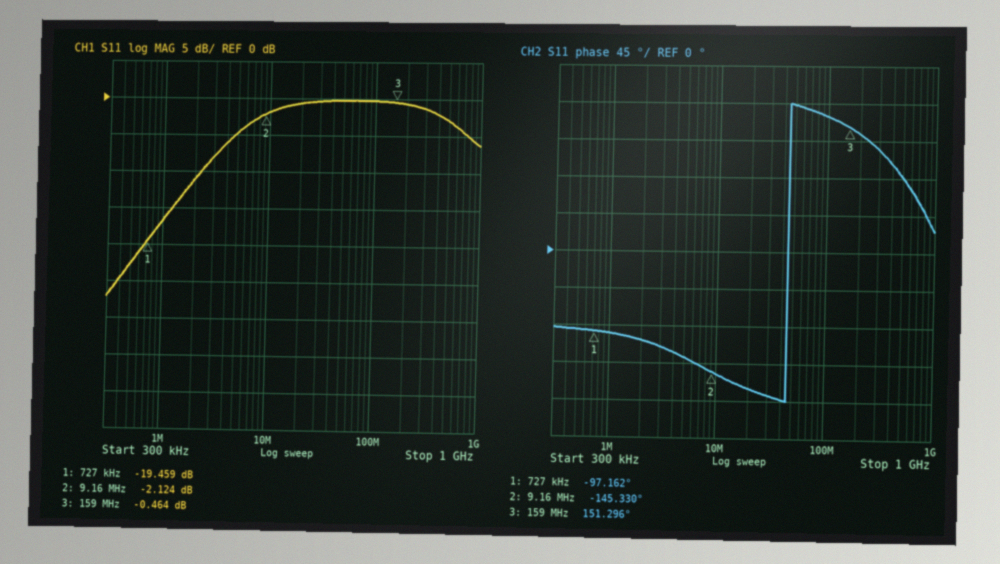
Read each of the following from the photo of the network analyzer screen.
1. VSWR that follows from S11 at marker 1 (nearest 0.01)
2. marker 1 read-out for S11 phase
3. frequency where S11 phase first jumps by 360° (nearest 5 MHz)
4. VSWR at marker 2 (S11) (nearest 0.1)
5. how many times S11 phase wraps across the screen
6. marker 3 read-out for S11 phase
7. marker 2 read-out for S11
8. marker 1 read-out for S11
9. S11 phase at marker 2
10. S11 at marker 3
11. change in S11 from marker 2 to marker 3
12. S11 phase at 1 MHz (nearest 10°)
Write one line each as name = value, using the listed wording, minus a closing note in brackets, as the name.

VSWR that follows from S11 at marker 1 = 1.24
marker 1 read-out for S11 phase = -97.162°
frequency where S11 phase first jumps by 360° = 45 MHz
VSWR at marker 2 (S11) = 8.2
how many times S11 phase wraps across the screen = 1
marker 3 read-out for S11 phase = 151.296°
marker 2 read-out for S11 = -2.124 dB
marker 1 read-out for S11 = -19.459 dB
S11 phase at marker 2 = -145.330°
S11 at marker 3 = -0.464 dB
change in S11 from marker 2 to marker 3 = 1.660 dB
S11 phase at 1 MHz = -100°
